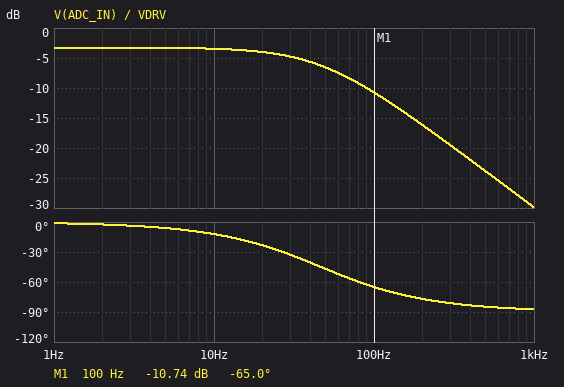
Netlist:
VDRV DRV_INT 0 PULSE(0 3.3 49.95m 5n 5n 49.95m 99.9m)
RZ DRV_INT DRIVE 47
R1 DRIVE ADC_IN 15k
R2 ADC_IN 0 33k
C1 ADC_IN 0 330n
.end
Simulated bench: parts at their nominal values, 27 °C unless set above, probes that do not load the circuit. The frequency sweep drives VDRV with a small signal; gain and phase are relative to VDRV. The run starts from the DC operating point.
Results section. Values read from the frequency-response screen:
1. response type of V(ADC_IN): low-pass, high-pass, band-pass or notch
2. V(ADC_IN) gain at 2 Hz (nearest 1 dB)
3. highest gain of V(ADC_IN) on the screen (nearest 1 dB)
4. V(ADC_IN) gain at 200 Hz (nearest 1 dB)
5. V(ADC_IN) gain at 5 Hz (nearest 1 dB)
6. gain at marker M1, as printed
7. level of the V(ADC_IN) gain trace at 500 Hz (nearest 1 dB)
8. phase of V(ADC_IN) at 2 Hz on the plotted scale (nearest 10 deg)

low-pass
-3 dB
-3 dB
-16 dB
-3 dB
-10.74 dB
-24 dB
0 deg
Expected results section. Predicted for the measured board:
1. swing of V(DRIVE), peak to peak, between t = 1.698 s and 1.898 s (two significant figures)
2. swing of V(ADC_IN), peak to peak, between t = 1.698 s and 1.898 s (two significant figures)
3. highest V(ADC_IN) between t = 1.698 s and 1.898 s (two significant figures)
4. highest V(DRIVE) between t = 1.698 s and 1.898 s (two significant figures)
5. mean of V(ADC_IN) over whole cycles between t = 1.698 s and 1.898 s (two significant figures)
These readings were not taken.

3.3 V
2.3 V
2.3 V
3.3 V
1.1 V
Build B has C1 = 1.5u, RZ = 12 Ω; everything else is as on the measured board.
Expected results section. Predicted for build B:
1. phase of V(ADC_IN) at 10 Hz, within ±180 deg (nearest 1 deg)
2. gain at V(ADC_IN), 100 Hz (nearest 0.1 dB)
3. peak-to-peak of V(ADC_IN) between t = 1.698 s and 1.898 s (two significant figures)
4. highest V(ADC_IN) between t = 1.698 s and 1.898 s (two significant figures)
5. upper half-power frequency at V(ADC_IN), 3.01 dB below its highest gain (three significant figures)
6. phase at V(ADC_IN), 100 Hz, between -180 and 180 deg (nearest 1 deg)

-44 deg
-23.1 dB
2.1 V
2.2 V
10.3 Hz
-84 deg
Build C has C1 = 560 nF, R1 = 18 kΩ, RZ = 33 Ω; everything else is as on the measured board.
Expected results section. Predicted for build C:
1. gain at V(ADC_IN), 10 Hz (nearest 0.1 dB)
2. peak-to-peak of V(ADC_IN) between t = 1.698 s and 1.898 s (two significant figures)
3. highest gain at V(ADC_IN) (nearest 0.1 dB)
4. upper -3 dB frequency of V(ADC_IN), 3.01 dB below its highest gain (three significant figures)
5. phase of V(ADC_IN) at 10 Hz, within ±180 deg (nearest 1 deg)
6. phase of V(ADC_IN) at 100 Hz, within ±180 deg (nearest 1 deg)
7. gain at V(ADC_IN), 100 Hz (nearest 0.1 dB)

-4.5 dB
2.1 V
-3.8 dB
24.4 Hz
-22 deg
-76 deg
-16.3 dB
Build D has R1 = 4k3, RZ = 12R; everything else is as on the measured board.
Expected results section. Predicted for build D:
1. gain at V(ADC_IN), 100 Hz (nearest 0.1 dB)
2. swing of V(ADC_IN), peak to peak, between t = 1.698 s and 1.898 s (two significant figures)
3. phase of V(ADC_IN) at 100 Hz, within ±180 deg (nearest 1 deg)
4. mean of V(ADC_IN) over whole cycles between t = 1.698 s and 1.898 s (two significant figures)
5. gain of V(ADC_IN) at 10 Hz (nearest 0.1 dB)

-3.2 dB
2.9 V
-38 deg
1.5 V
-1.1 dB
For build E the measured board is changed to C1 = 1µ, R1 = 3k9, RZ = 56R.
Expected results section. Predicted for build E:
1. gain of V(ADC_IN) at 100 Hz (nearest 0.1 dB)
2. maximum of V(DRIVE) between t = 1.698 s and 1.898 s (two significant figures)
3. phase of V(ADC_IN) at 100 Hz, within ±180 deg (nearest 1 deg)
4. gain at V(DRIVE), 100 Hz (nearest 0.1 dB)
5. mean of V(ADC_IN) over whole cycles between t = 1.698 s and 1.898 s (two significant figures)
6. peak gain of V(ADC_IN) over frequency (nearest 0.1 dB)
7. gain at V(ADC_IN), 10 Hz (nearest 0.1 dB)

-8.7 dB
3.3 V
-66 deg
-0.1 dB
1.5 V
-1.0 dB
-1.2 dB
